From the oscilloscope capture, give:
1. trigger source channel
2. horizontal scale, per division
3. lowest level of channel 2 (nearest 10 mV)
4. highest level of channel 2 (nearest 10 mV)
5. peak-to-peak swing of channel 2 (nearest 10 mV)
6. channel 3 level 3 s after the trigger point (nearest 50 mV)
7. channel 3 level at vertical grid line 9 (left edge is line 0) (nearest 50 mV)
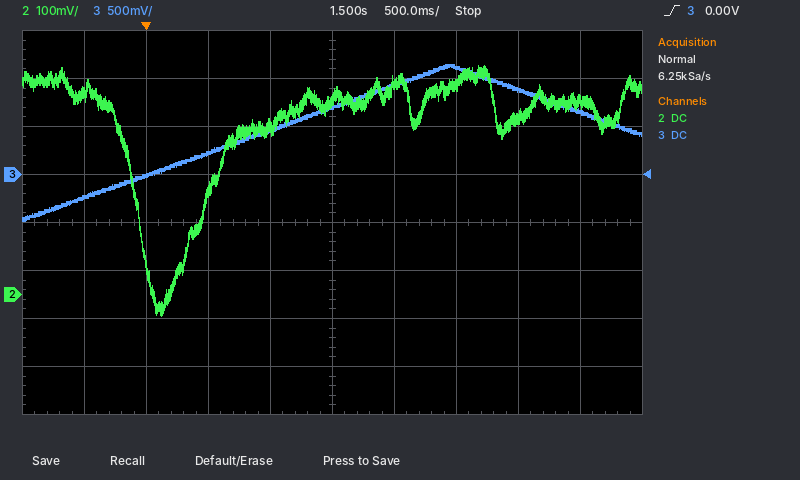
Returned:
channel 3
500 ms
-40 mV
480 mV
520 mV
900 mV
650 mV
